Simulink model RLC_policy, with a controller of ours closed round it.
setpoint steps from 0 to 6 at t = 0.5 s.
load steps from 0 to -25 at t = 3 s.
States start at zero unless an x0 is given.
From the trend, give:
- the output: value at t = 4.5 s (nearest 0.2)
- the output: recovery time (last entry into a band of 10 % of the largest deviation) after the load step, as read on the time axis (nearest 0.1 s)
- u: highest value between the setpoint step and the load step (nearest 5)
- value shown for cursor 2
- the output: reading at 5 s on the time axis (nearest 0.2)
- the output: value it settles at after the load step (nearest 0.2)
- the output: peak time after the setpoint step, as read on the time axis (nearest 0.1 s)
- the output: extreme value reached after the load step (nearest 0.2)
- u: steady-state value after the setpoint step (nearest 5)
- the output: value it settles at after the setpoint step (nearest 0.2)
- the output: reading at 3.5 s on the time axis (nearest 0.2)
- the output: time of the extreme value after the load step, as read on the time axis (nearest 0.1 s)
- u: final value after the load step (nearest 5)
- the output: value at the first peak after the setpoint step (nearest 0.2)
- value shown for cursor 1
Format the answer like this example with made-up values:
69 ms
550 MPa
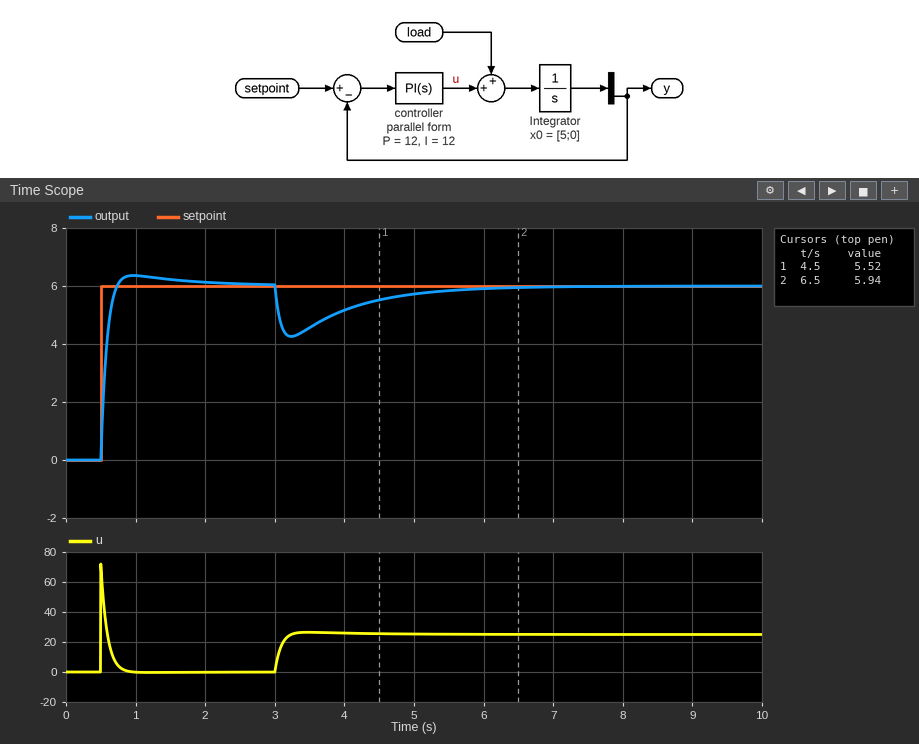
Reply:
5.6
5.4 s
70
5.94
5.8
6.0
1.0 s
4.2
0
6.0
4.6
3.2 s
25
6.4
5.52
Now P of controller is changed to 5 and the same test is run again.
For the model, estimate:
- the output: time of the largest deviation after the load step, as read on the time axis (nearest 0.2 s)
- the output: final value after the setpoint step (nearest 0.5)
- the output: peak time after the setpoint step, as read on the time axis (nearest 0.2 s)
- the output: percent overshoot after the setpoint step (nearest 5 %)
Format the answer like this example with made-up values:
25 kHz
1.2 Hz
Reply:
3.4 s
6.0
1.2 s
20 %
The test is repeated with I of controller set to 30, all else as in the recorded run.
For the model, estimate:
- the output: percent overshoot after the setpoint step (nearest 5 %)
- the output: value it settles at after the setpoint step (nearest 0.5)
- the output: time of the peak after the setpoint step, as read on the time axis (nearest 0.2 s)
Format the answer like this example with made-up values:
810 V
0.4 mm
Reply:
10 %
6.0
0.8 s
